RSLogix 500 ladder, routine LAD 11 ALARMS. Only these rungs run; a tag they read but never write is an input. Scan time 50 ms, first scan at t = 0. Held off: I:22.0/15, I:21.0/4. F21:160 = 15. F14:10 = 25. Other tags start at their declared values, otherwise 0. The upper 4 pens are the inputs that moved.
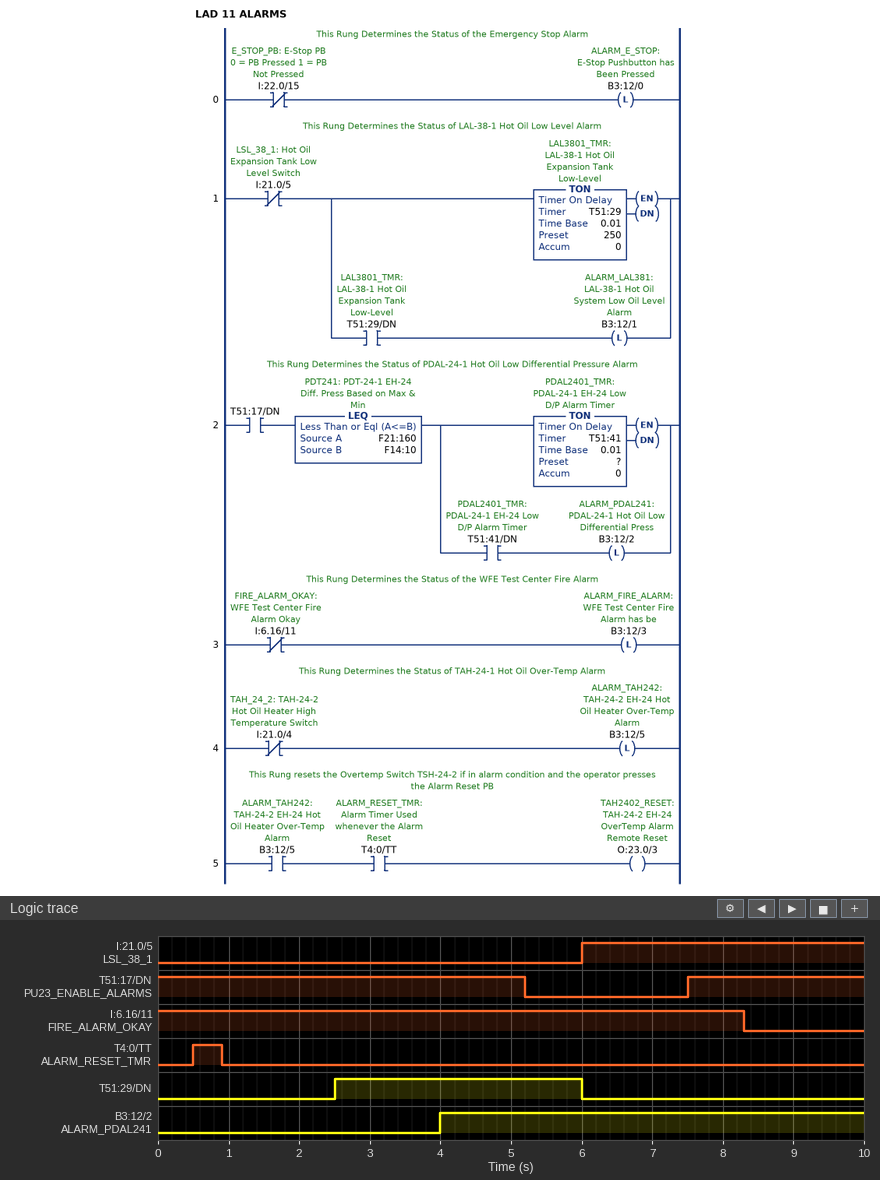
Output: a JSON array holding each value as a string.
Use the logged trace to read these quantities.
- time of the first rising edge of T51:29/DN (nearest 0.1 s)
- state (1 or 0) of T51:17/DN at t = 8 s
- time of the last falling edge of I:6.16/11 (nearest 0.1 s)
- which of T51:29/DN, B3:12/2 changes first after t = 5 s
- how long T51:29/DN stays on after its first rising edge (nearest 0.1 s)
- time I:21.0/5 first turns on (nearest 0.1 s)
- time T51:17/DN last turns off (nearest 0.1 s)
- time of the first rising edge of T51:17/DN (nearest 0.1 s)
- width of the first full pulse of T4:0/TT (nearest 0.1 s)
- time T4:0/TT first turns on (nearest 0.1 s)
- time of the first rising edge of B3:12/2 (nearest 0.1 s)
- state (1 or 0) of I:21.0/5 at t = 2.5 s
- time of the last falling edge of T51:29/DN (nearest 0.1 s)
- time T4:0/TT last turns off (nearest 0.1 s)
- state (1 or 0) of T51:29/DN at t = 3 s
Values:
["2.5 s", "1", "8.3 s", "T51:29/DN", "3.5 s", "6.0 s", "5.2 s", "7.5 s", "0.4 s", "0.5 s", "4.0 s", "0", "6.0 s", "0.9 s", "1"]
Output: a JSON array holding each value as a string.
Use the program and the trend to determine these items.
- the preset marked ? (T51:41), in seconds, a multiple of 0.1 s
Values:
["4.0 s"]
